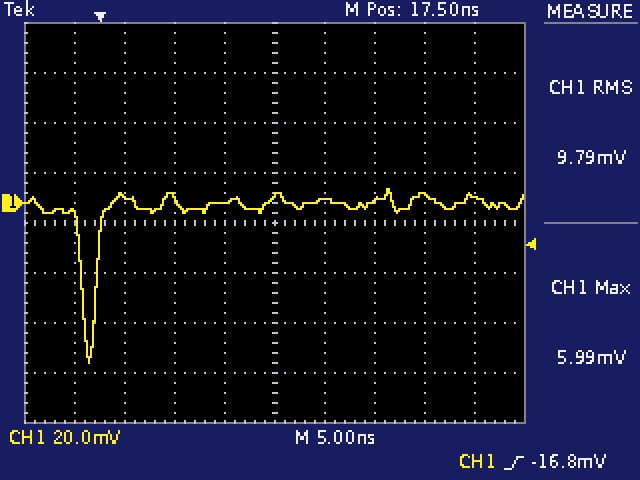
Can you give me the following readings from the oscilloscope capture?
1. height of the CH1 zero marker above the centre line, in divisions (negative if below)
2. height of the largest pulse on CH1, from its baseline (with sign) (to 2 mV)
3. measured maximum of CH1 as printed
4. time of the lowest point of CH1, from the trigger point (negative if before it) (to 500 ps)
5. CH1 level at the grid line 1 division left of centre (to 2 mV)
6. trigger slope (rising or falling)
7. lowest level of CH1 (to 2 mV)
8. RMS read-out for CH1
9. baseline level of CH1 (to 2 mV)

+0.4 div
-64 mV
5.99 mV
-1.0 ns
0 mV
rising
-64 mV
9.79 mV
0 mV
